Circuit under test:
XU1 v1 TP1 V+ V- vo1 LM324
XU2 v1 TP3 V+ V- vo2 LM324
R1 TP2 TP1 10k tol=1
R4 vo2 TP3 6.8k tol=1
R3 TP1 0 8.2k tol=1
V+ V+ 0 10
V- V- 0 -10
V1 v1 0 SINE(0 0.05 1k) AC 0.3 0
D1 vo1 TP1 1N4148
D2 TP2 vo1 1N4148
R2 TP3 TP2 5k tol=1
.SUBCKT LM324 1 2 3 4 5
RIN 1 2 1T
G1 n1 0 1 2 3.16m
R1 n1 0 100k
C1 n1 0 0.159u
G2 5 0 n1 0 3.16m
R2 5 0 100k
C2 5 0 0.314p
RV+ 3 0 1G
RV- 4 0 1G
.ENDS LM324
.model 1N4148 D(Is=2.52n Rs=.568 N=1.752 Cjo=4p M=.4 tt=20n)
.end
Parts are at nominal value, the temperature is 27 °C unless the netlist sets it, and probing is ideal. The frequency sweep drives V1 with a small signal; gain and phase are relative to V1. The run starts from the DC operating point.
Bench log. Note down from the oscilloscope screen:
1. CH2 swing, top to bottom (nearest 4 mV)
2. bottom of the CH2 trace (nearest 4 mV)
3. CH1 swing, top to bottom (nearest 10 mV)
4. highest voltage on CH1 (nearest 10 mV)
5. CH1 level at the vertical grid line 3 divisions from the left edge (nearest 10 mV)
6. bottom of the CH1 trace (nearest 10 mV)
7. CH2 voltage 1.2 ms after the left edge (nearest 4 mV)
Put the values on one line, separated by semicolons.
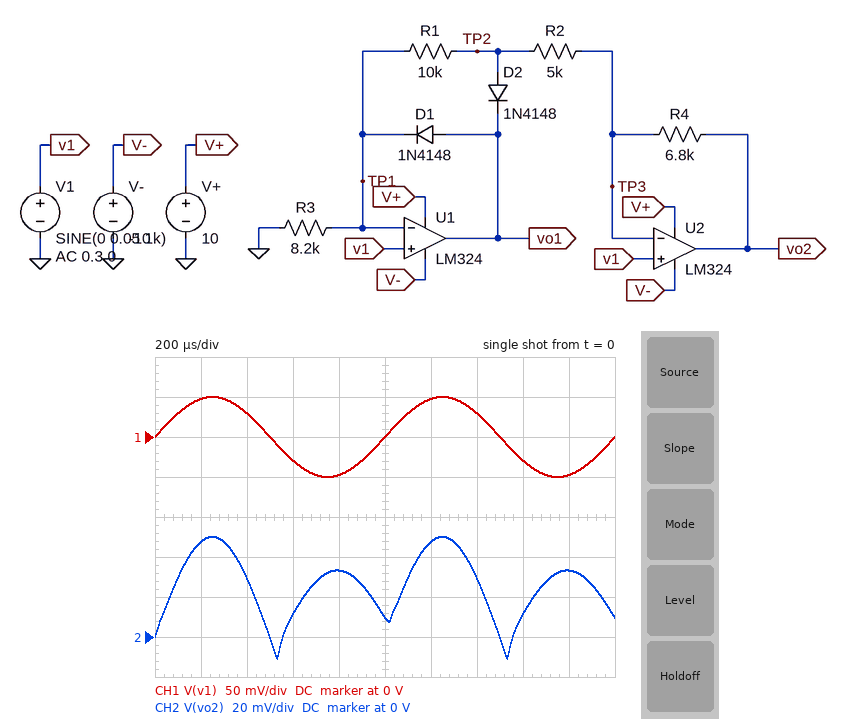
60 mV; -12 mV; 100 mV; 50 mV; -30 mV; -50 mV; 48 mV
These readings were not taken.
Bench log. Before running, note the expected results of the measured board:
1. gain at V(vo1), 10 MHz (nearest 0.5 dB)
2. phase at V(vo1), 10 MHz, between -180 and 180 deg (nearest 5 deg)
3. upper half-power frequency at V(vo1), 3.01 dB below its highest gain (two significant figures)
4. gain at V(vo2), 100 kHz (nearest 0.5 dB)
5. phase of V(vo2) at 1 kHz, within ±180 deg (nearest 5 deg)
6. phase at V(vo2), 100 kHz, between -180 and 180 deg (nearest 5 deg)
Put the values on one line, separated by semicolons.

-37.0 dB; -125 deg; 340 Hz; 1.0 dB; 10 deg; -20 deg
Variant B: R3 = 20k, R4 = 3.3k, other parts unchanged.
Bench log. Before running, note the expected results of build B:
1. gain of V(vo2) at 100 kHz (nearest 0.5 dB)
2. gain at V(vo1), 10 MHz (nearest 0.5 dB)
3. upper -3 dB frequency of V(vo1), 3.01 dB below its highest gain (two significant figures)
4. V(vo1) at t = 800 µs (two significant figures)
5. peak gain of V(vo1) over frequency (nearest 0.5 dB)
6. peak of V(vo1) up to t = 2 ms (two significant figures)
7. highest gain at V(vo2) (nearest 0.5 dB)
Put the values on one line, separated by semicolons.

0 dB; -32.5 dB; 500 Hz; -430 mV; 56.5 dB; 360 mV; 0.5 dB
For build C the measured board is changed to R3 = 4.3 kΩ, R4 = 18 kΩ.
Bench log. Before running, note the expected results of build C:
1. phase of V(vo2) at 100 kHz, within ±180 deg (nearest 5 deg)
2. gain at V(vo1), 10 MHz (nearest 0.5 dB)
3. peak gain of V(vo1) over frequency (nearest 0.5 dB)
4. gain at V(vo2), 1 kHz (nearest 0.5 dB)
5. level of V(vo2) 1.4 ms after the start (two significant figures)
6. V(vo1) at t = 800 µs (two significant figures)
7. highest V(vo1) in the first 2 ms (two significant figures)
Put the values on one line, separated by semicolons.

-25 deg; -41.0 dB; 69.5 dB; 4.0 dB; 28 mV; -590 mV; 430 mV
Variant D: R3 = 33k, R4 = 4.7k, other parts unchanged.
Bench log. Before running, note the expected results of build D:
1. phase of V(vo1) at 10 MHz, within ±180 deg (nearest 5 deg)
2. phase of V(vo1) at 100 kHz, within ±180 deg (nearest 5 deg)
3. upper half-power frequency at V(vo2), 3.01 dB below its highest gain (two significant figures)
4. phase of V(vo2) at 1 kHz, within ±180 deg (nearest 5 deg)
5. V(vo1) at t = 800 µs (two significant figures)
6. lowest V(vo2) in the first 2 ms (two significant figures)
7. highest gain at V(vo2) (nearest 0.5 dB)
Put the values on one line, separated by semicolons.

-130 deg; -80 deg; 480 kHz; 5 deg; -400 mV; -36 mV; 0.5 dB
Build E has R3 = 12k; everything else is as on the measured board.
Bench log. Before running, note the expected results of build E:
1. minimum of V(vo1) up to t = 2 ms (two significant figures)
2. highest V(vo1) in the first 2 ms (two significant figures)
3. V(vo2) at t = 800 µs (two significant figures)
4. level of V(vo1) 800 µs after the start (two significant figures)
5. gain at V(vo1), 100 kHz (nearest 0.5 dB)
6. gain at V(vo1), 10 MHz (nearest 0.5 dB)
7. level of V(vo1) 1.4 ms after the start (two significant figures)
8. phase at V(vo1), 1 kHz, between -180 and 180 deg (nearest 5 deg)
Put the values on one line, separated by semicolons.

-480 mV; 390 mV; 7.6 mV; -470 mV; 13.0 dB; -35.0 dB; 340 mV; -70 deg
